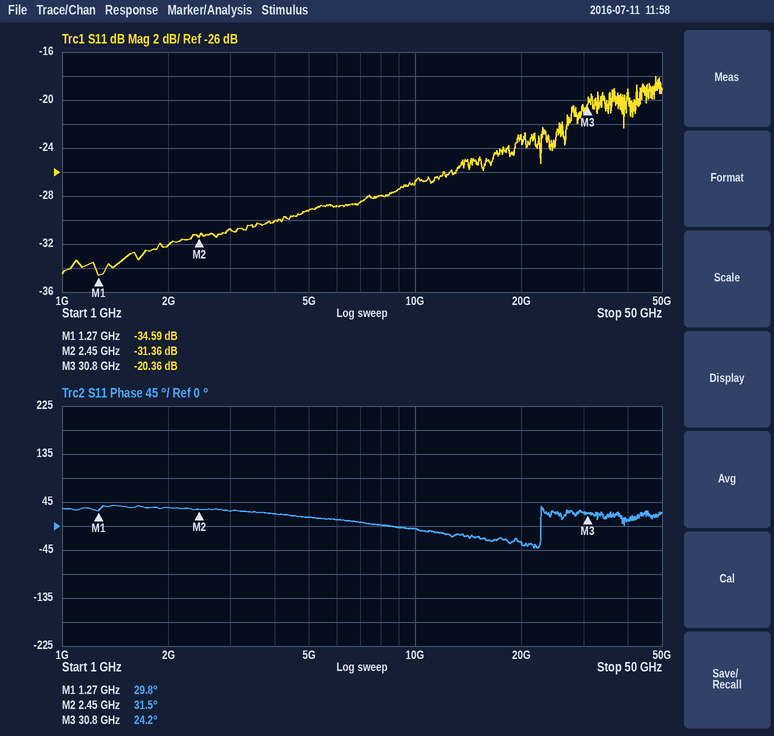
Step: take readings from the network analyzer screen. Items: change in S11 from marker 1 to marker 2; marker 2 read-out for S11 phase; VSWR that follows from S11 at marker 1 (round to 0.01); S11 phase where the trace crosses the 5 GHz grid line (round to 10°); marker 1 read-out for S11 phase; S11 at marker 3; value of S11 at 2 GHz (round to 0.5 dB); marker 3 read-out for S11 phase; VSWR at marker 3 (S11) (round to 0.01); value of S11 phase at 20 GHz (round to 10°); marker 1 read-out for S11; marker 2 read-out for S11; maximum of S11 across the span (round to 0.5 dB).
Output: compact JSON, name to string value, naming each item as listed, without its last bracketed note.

{"change in S11 from marker 1 to marker 2": "3.23 dB", "marker 2 read-out for S11 phase": "31.5°", "VSWR that follows from S11 at marker 1": "1.04", "S11 phase where the trace crosses the 5 GHz grid line": "20°", "marker 1 read-out for S11 phase": "29.8°", "S11 at marker 3": "-20.36 dB", "value of S11 at 2 GHz": "-32.0 dB", "marker 3 read-out for S11 phase": "24.2°", "VSWR at marker 3 (S11)": "1.21", "value of S11 phase at 20 GHz": "-30°", "marker 1 read-out for S11": "-34.59 dB", "marker 2 read-out for S11": "-31.36 dB", "maximum of S11 across the span": "-18.0 dB"}
